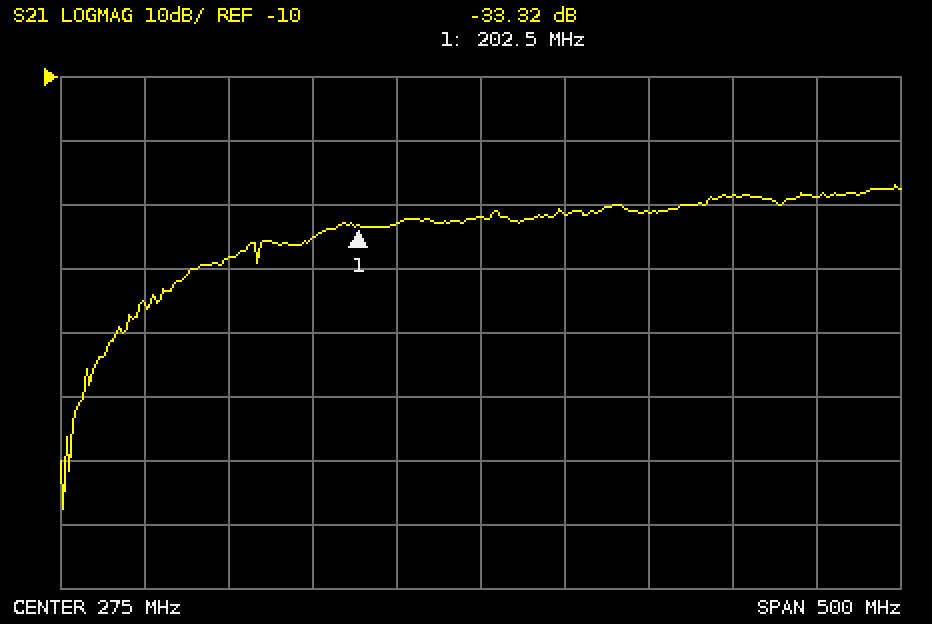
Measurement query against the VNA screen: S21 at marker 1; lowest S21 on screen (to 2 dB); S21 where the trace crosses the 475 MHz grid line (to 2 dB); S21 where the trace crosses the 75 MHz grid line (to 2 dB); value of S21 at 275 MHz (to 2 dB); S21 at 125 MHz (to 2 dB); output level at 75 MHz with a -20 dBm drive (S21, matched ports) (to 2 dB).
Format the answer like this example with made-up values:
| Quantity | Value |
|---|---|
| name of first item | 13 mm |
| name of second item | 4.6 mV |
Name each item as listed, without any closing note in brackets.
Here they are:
| Quantity | Value |
|---|---|
| S21 at marker 1 | -33.32 dB |
| lowest S21 on screen | -78 dB |
| S21 where the trace crosses the 475 MHz grid line | -28 dB |
| S21 where the trace crosses the 75 MHz grid line | -46 dB |
| value of S21 at 275 MHz | -32 dB |
| S21 at 125 MHz | -38 dB |
| output level at 75 MHz with a -20 dBm drive (S21, matched ports) | -66 dBm |
